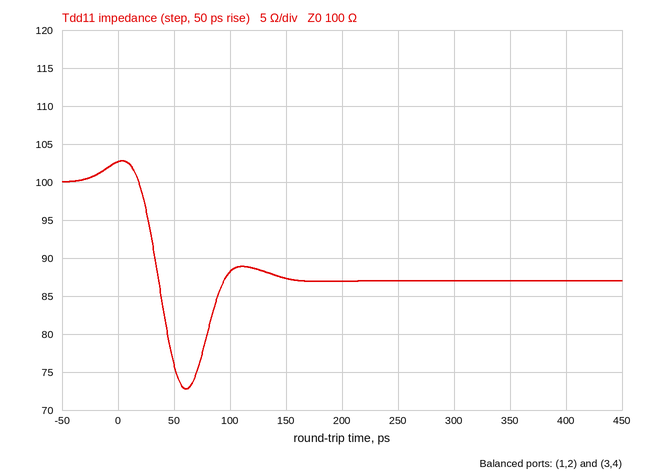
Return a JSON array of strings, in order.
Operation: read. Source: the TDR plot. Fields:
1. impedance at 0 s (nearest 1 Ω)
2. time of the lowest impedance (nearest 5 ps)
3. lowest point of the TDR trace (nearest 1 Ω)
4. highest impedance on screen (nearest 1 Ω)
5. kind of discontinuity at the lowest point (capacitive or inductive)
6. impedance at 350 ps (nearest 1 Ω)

["103 Ω", "60 ps", "73 Ω", "103 Ω", "capacitive", "87 Ω"]
